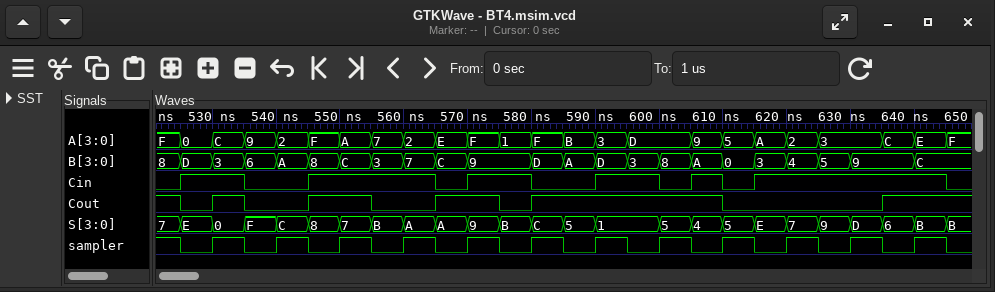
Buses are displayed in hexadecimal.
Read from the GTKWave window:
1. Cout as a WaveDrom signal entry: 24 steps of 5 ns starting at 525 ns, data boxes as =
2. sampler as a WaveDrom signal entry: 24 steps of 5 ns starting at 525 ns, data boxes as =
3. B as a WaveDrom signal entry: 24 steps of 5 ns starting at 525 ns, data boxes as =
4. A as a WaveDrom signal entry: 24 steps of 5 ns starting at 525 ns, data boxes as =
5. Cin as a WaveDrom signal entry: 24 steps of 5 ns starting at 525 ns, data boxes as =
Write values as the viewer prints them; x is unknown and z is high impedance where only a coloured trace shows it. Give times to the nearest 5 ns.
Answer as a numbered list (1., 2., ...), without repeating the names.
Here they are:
1. {name: 'Cout', wave: '010.1.0.1.01.....0....1.'}
2. {name: 'sampler', wave: '010101010101010101010101'}
3. {name: 'B', wave: '==========.===========.=', data: 'D 3 6 A 8 C 3 7 C 9 D A D 3 8 A 0 3 4 5 9 C'}
4. {name: 'A', wave: '===============.=====.==', data: '0 C 9 2 F A 7 2 E F 1 F B 3 D 9 5 A 2 3 C E'}
5. {name: 'Cin', wave: '1.0.1...01.0.1.0101.....'}
